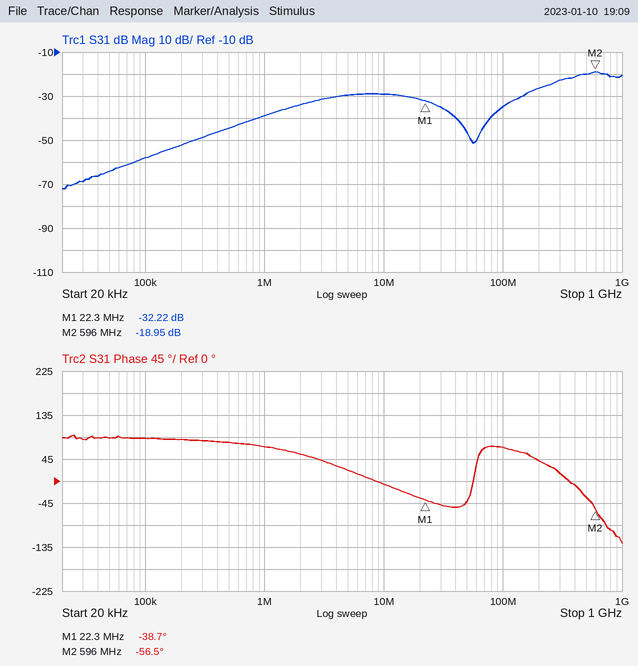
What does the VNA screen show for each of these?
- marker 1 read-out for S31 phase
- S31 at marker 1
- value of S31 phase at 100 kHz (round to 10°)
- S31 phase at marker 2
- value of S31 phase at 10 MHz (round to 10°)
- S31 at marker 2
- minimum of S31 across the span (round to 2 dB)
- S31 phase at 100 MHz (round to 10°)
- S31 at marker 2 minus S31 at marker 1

-38.7°
-32.22 dB
90°
-56.5°
-10°
-18.95 dB
-72 dB
70°
13.27 dB
